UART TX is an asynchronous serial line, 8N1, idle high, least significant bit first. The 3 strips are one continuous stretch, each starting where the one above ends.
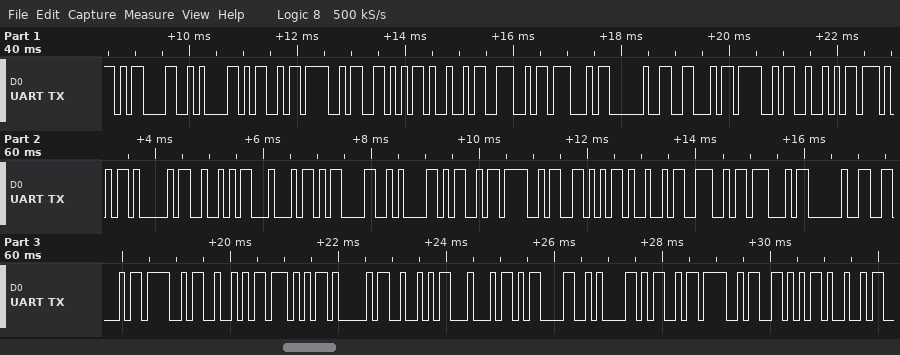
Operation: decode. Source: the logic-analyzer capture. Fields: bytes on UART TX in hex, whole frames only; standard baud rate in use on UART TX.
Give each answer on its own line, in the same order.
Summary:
0D 0A 4D 4F 56 49 4E 47 20 46 4F 52 57 41 52 44 0D 0A 4D 4F 56 49 4E 47 20 46 4F 52 57 41 52 44 0D 0A 4D 4F 56 49
9600 baud
